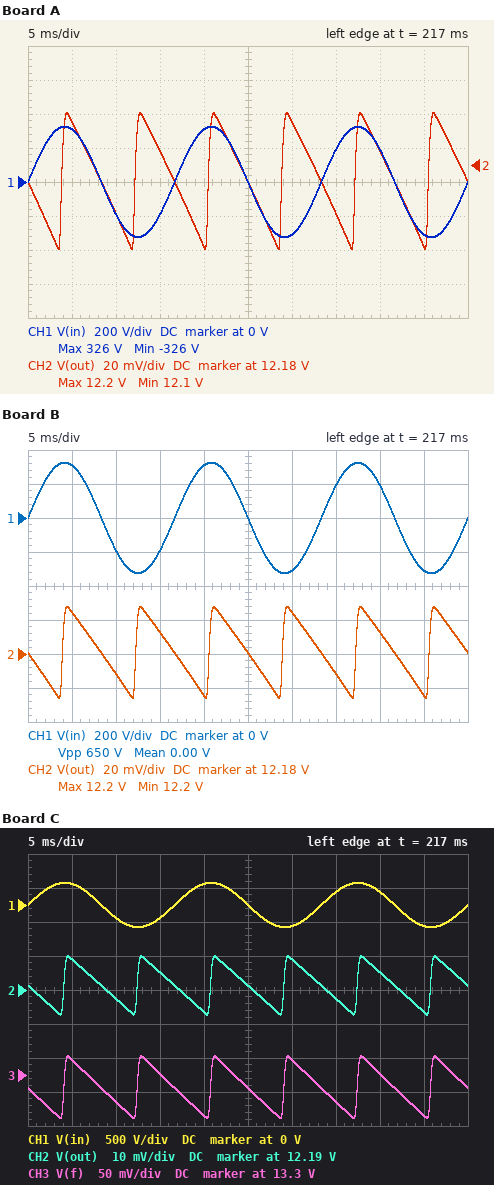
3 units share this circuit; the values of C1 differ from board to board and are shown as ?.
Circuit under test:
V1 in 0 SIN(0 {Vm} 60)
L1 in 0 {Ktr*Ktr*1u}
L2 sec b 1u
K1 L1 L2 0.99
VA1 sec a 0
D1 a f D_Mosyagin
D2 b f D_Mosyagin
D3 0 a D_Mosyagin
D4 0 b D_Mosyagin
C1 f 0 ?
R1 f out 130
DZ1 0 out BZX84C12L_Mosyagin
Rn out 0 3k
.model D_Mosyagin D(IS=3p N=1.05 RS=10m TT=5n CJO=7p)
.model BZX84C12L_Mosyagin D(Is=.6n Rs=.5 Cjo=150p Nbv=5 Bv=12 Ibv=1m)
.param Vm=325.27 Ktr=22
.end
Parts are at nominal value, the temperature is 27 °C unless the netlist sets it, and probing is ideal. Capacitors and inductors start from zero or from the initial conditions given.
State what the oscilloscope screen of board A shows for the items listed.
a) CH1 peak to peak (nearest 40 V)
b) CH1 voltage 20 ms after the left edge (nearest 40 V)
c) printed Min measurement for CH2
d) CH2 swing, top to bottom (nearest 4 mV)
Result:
640 V
320 V
12.1 V
80 mV
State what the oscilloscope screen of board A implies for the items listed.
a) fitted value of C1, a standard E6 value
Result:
150 µF
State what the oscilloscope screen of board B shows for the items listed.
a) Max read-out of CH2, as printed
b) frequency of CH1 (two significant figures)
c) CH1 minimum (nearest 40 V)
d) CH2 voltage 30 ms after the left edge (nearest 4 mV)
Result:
12.2 V
60 Hz
-320 V
12.204 V
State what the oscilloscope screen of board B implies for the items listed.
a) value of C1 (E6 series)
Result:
220 µF
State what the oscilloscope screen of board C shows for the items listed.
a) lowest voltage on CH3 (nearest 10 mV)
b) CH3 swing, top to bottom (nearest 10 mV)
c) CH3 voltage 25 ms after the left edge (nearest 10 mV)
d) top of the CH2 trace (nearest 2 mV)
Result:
13.24 V
90 mV
13.28 V
12.200 V
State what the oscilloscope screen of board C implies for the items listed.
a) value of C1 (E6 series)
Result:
680 µF
